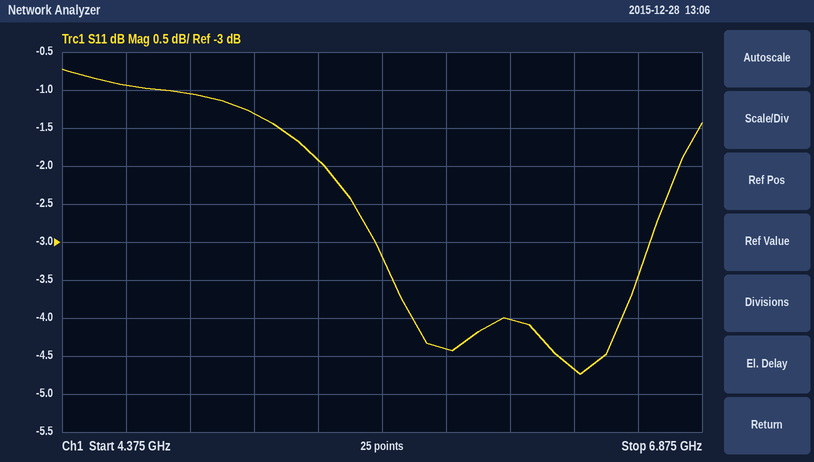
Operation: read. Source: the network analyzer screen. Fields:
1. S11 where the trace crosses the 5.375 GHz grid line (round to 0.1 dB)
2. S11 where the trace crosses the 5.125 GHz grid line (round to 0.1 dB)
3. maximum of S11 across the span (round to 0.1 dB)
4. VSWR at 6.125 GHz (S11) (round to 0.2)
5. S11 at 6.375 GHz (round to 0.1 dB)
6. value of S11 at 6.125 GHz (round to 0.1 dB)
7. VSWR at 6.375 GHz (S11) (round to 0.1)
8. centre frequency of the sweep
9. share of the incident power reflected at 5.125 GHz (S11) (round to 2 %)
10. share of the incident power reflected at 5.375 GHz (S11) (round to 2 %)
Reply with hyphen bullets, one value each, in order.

- -1.9 dB
- -1.3 dB
- -0.7 dB
- 4.4
- -4.7 dB
- -4.0 dB
- 3.8
- 5.625 GHz
- 74 %
- 64 %
